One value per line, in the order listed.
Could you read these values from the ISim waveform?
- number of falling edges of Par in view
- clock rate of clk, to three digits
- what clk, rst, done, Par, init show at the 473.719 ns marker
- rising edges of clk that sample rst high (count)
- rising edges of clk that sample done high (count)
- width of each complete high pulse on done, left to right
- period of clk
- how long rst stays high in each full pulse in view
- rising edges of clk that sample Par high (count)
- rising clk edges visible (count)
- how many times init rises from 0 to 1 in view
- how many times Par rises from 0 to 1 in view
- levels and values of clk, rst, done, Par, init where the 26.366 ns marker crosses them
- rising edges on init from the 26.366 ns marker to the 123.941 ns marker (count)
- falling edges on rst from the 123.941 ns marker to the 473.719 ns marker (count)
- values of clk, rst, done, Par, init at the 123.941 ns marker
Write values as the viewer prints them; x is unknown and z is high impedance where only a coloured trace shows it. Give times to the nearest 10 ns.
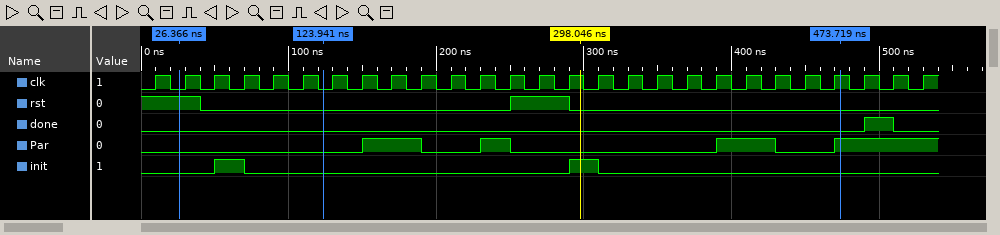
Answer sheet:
3
50.0 MHz
clk=1, rst=0, done=0, Par=1, init=0
4
1
20 ns
20 ns
40 ns
8
27
2
4
clk=0, rst=1, done=0, Par=0, init=0
1
1
clk=0, rst=0, done=0, Par=0, init=0
